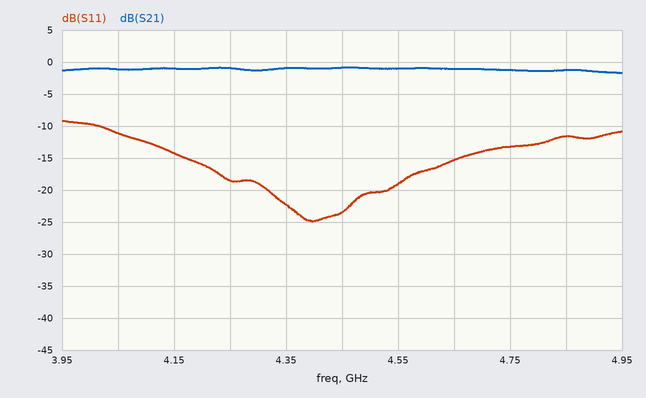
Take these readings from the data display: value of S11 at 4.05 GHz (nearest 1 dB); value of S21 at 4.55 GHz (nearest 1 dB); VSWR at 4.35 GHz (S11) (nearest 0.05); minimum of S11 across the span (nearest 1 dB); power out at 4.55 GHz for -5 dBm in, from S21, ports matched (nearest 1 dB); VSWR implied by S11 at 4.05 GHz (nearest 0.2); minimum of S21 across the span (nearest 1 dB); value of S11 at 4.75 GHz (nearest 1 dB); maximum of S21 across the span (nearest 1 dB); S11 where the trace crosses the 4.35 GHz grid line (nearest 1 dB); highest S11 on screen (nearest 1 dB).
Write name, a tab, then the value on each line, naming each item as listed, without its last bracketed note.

value of S11 at 4.05 GHz	-11 dB
value of S21 at 4.55 GHz	-1 dB
VSWR at 4.35 GHz (S11)	1.15
minimum of S11 across the span	-25 dB
power out at 4.55 GHz for -5 dBm in, from S21, ports matched	-6 dBm
VSWR implied by S11 at 4.05 GHz	1.8
minimum of S21 across the span	-2 dB
value of S11 at 4.75 GHz	-13 dB
maximum of S21 across the span	-1 dB
S11 where the trace crosses the 4.35 GHz grid line	-22 dB
highest S11 on screen	-9 dB
